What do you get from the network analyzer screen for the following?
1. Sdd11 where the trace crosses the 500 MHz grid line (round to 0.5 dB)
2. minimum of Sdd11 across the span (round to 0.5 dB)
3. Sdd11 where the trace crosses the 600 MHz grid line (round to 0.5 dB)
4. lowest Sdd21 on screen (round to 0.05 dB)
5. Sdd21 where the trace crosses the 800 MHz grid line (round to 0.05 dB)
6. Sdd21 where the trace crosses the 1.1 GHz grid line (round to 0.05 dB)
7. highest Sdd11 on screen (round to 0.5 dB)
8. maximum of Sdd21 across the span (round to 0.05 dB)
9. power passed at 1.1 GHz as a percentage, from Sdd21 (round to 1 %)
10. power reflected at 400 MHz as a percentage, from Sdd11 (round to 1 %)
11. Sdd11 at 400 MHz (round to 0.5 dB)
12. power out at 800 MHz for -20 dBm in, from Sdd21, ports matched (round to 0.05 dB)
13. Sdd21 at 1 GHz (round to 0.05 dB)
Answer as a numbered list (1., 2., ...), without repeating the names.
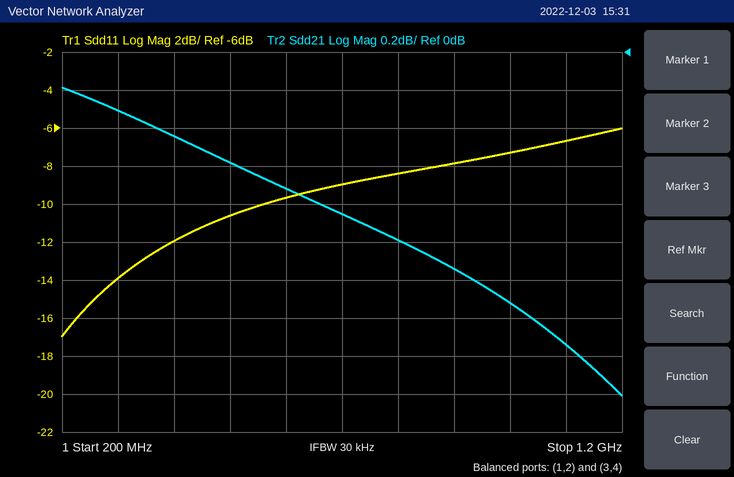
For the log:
1. -10.5 dB
2. -17.0 dB
3. -9.5 dB
4. -1.80 dB
5. -1.00 dB
6. -1.55 dB
7. -6.0 dB
8. -0.20 dB
9. 70 %
10. 6 %
11. -12.0 dB
12. -21.00 dBm
13. -1.30 dB
